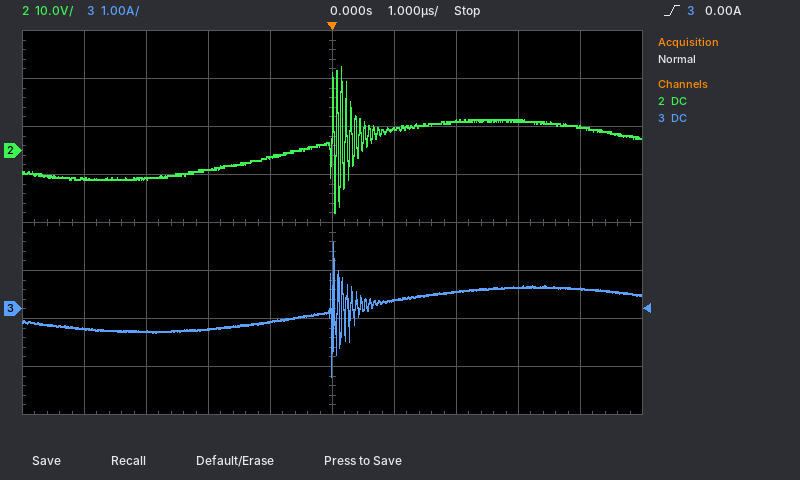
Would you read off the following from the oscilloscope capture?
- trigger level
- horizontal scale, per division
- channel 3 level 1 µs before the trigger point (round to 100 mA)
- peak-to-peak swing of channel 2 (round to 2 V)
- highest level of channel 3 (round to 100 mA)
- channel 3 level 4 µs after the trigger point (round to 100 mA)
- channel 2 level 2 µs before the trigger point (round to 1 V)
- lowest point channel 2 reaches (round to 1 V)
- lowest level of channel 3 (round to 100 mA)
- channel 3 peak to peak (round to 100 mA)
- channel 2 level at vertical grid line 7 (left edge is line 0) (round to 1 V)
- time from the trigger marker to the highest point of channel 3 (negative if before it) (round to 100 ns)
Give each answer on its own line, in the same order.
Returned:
0.00 A
1 µs
-300 mA
30 V
1.4 A
400 mA
-4 V
-13 V
-1.4 A
2.8 A
6 V
0.0 µs
